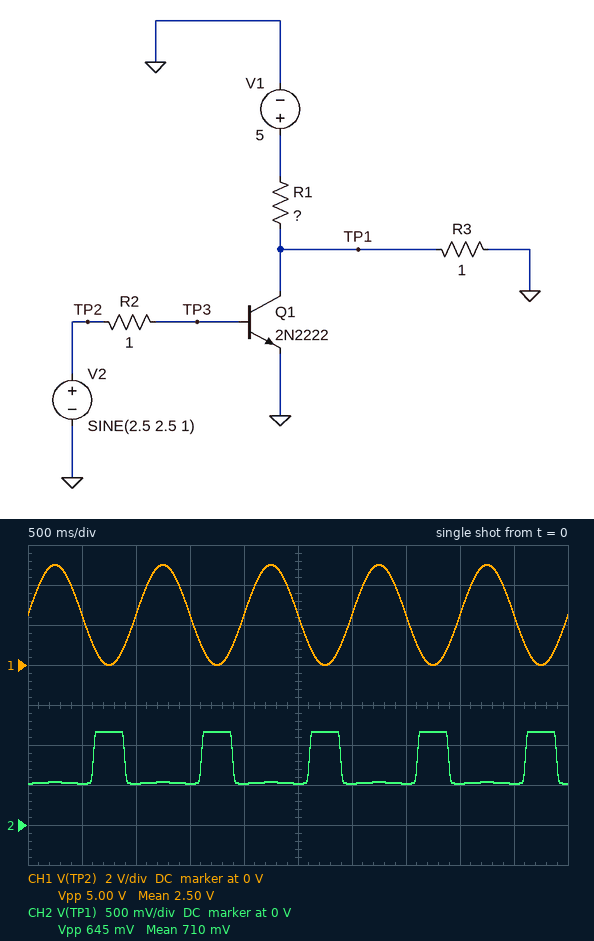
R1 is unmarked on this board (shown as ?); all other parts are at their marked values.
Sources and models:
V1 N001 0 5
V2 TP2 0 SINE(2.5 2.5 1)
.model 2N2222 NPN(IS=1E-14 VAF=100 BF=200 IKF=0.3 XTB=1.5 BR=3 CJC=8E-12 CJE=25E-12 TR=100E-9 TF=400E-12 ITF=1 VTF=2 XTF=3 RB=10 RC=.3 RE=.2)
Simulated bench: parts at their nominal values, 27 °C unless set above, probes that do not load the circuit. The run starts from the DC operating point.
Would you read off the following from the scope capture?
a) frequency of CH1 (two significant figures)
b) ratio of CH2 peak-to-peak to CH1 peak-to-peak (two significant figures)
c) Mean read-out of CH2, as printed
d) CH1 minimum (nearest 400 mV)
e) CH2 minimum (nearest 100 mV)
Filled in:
1.0 Hz
0.13
710 mV
0 V
500 mV
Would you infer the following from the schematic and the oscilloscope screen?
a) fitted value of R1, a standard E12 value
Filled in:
3.3 Ω
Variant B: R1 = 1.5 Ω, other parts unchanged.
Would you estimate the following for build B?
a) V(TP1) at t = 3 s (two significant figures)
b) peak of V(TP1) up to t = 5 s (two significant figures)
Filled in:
980 mV
2.0 V
